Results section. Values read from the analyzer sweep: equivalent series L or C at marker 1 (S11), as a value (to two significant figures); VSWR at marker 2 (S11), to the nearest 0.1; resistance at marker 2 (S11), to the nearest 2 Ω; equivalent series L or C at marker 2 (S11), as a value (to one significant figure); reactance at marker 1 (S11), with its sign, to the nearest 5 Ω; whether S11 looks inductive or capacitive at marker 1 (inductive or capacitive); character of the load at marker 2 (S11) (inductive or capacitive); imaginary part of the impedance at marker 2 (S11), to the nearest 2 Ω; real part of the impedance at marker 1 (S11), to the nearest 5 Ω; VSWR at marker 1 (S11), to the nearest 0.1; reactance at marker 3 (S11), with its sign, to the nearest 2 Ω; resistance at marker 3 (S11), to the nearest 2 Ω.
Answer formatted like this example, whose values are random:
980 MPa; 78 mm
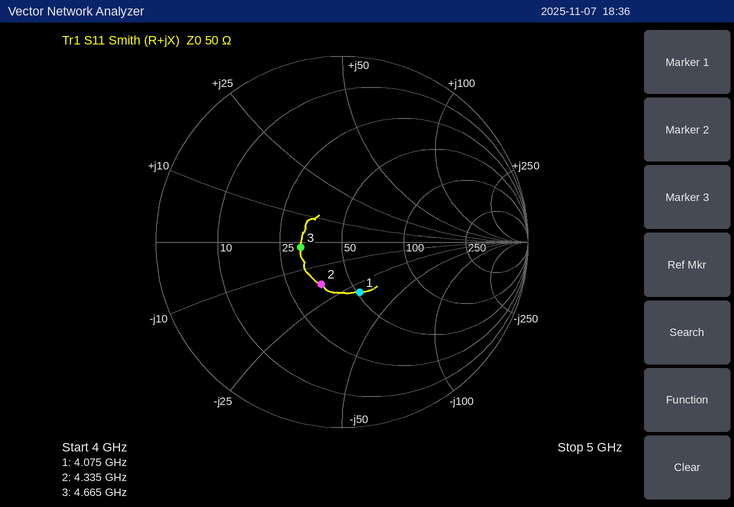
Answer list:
1.3 pF; 1.7; 36 Ω; 2 pF; -30 Ω; capacitive; capacitive; -18 Ω; 50 Ω; 1.8; -2 Ω; 32 Ω
